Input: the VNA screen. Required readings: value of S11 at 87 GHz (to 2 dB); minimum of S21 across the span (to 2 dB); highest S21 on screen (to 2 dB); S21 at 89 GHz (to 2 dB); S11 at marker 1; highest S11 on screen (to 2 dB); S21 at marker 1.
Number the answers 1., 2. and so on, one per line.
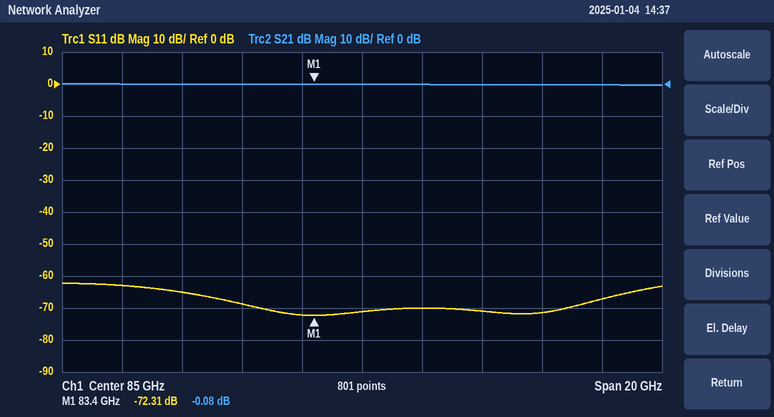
1. -70 dB
2. 0 dB
3. 0 dB
4. 0 dB
5. -72.31 dB
6. -62 dB
7. -0.08 dB
